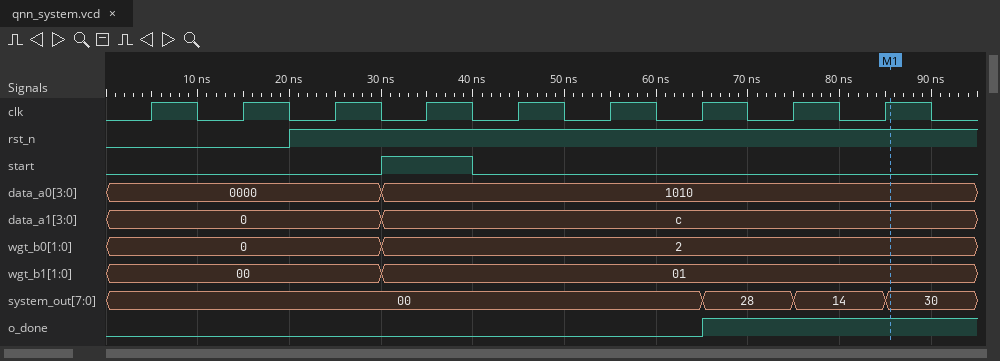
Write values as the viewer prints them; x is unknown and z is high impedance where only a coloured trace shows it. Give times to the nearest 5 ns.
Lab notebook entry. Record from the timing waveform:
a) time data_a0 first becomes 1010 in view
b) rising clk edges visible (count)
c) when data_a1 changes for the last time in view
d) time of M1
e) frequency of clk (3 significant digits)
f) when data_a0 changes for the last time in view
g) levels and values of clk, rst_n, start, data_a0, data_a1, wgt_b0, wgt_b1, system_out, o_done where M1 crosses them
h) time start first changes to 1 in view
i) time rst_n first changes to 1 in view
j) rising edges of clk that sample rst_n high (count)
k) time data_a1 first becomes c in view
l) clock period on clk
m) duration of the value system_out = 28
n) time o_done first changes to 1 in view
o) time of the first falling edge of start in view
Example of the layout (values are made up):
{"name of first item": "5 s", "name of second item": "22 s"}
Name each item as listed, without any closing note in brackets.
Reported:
{"time data_a0 first becomes 1010 in view": "30 ns", "rising clk edges visible": "9", "when data_a1 changes for the last time in view": "30 ns", "time of M1": "85 ns", "frequency of clk": "100 MHz", "when data_a0 changes for the last time in view": "30 ns", "levels and values of clk, rst_n, start, data_a0, data_a1, wgt_b0, wgt_b1, system_out, o_done where M1 crosses them": "clk=1, rst_n=1, start=0, data_a0=1010, data_a1=c, wgt_b0=2, wgt_b1=01, system_out=30, o_done=1", "time start first changes to 1 in view": "30 ns", "time rst_n first changes to 1 in view": "20 ns", "rising edges of clk that sample rst_n high": "7", "time data_a1 first becomes c in view": "30 ns", "clock period on clk": "10 ns", "duration of the value system_out = 28": "10 ns", "time o_done first changes to 1 in view": "65 ns", "time of the first falling edge of start in view": "40 ns"}
